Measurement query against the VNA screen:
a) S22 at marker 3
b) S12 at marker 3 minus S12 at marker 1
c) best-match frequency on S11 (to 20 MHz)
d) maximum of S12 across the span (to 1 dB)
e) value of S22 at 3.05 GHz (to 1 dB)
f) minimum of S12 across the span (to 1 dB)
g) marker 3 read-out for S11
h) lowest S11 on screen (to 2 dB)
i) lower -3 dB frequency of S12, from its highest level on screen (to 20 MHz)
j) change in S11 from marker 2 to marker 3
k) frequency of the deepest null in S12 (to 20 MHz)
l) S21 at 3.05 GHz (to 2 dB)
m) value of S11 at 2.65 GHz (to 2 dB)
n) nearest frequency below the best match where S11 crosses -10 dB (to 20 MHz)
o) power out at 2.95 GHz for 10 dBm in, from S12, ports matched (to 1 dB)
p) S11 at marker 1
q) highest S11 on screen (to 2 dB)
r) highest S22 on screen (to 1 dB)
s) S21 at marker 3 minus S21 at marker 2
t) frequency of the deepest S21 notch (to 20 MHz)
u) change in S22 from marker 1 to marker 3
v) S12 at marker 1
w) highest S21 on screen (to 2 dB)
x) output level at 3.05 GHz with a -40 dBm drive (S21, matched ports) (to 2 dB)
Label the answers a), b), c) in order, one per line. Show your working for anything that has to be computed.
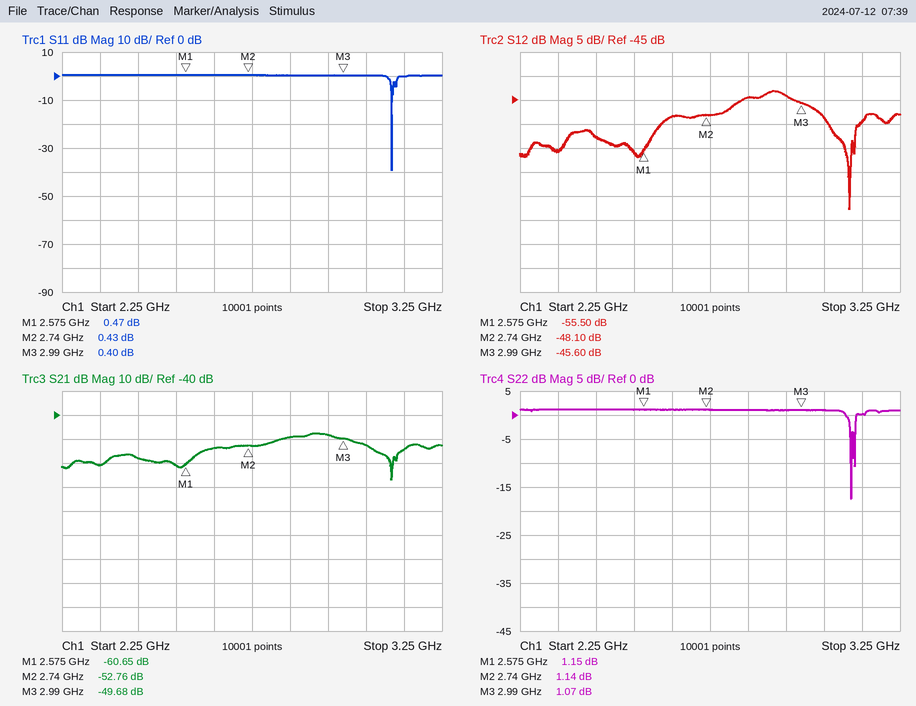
a) 1.07 dB
b) -45.6 − (-55.5) = 9.90 dB
c) 3.12 GHz
d) -43 dB
e) 1 dB
f) -68 dB
g) 0.40 dB
h) -40 dB
i) 2.82 GHz
j) 0.4 − (0.43) = -0.03 dB
k) 3.12 GHz
l) -52 dB
m) 0 dB
n) 3.12 GHz
o) 10 dBm + (-44 dB) = -34 dBm
p) 0.47 dB
q) 0 dB
r) 1 dB
s) -49.68 − (-52.76) = 3.08 dB
t) 3.12 GHz
u) 1.07 − (1.15) = -0.08 dB
v) -55.50 dB
w) -48 dB
x) -40 dBm + (-52 dB) = -92 dBm
